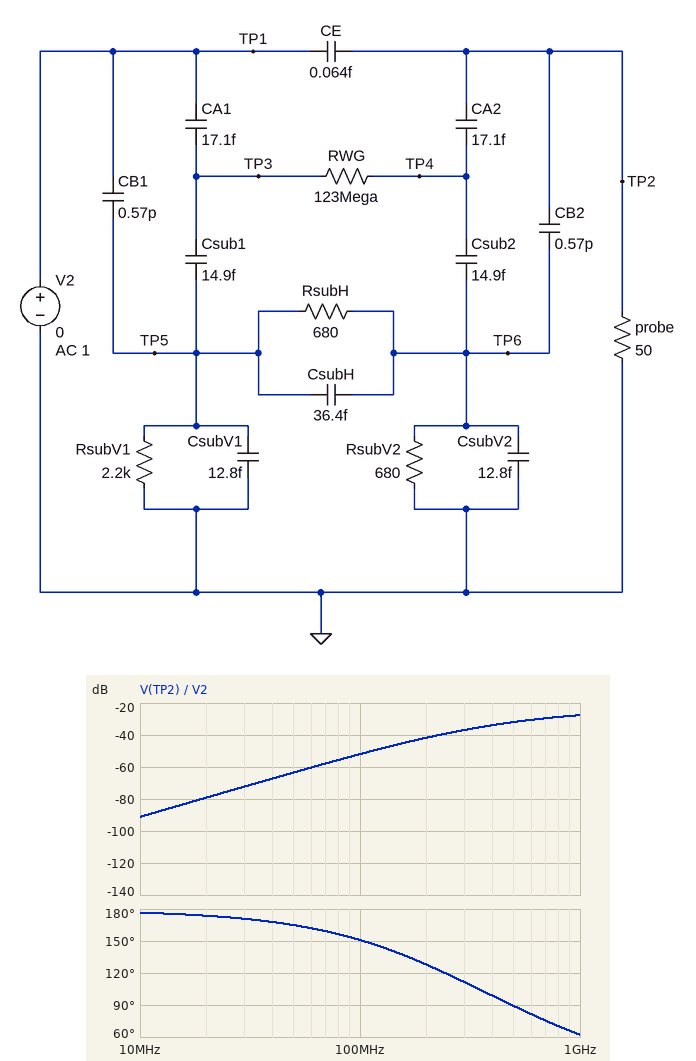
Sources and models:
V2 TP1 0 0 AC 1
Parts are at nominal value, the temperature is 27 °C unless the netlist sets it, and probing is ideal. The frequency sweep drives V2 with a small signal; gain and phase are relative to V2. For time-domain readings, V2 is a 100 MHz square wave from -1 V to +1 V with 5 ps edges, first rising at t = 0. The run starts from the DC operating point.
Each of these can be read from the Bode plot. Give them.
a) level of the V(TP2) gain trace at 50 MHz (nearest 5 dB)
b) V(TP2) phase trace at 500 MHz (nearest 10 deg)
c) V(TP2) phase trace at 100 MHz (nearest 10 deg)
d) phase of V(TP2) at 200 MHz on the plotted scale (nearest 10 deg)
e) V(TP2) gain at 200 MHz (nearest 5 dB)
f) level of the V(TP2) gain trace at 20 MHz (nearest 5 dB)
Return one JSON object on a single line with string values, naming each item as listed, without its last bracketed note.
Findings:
{"level of the V(TP2) gain trace at 50 MHz": "-65 dB", "V(TP2) phase trace at 500 MHz": "90 deg", "V(TP2) phase trace at 100 MHz": "150 deg", "phase of V(TP2) at 200 MHz on the plotted scale": "130 deg", "V(TP2) gain at 200 MHz": "-40 dB", "level of the V(TP2) gain trace at 20 MHz": "-80 dB"}
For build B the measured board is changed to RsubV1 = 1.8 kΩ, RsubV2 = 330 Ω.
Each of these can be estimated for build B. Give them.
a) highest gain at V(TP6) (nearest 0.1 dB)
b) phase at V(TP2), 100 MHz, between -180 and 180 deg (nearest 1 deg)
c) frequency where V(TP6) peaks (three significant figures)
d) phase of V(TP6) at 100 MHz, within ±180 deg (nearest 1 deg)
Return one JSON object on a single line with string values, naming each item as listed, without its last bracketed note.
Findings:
{"highest gain at V(TP6)": "-13.7 dB", "phase at V(TP2), 100 MHz, between -180 and 180 deg": "160 deg", "frequency where V(TP6) peaks": "634 MHz", "phase of V(TP6) at 100 MHz, within ±180 deg": "71 deg"}
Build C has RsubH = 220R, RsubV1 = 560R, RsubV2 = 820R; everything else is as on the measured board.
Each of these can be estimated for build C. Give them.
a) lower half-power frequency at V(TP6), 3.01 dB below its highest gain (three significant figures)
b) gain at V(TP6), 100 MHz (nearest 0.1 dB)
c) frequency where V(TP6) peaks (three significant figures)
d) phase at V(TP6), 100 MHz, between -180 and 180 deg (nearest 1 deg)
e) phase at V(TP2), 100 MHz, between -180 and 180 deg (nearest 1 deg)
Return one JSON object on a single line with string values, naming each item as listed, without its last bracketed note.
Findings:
{"lower half-power frequency at V(TP6), 3.01 dB below its highest gain": "301 MHz", "gain at V(TP6), 100 MHz": "-19.9 dB", "frequency where V(TP6) peaks": "971 MHz", "phase at V(TP6), 100 MHz, between -180 and 180 deg": "74 deg", "phase at V(TP2), 100 MHz, between -180 and 180 deg": "163 deg"}
